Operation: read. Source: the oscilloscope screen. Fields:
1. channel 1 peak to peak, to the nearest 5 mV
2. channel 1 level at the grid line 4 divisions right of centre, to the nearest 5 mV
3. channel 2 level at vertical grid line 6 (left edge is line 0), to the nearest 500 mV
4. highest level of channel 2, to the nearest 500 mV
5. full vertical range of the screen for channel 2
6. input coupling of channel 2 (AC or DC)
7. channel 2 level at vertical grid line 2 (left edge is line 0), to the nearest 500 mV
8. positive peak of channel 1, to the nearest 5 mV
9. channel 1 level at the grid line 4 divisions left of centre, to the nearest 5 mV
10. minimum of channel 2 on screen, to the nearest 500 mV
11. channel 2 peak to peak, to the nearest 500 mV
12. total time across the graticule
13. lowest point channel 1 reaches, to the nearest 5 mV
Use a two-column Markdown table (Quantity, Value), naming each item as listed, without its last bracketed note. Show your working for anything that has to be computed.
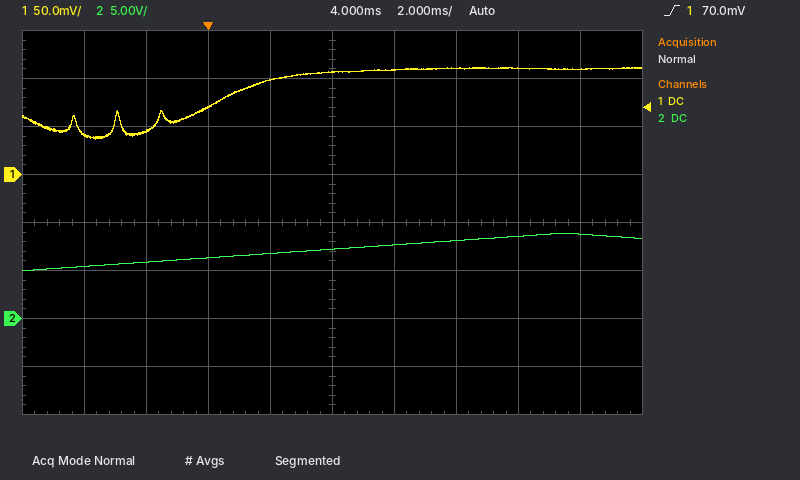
| Quantity | Value |
|---|---|
| channel 1 peak to peak, to the nearest 5 mV | 110 mV − (35 mV) = 75 mV |
| channel 1 level at the grid line 4 divisions right of centre, to the nearest 5 mV | 110 mV |
| channel 2 level at vertical grid line 6 (left edge is line 0), to the nearest 500 mV | 7.5 V |
| highest level of channel 2, to the nearest 500 mV | 9.0 V |
| full vertical range of the screen for channel 2 | 40 V |
| input coupling of channel 2 | DC |
| channel 2 level at vertical grid line 2 (left edge is line 0), to the nearest 500 mV | 6.0 V |
| positive peak of channel 1, to the nearest 5 mV | 110 mV |
| channel 1 level at the grid line 4 divisions left of centre, to the nearest 5 mV | 40 mV |
| minimum of channel 2 on screen, to the nearest 500 mV | 5.0 V |
| channel 2 peak to peak, to the nearest 500 mV | 9.0 V − (5.0 V) = 4.0 V |
| total time across the graticule | 20 ms |
| lowest point channel 1 reaches, to the nearest 5 mV | 35 mV |
